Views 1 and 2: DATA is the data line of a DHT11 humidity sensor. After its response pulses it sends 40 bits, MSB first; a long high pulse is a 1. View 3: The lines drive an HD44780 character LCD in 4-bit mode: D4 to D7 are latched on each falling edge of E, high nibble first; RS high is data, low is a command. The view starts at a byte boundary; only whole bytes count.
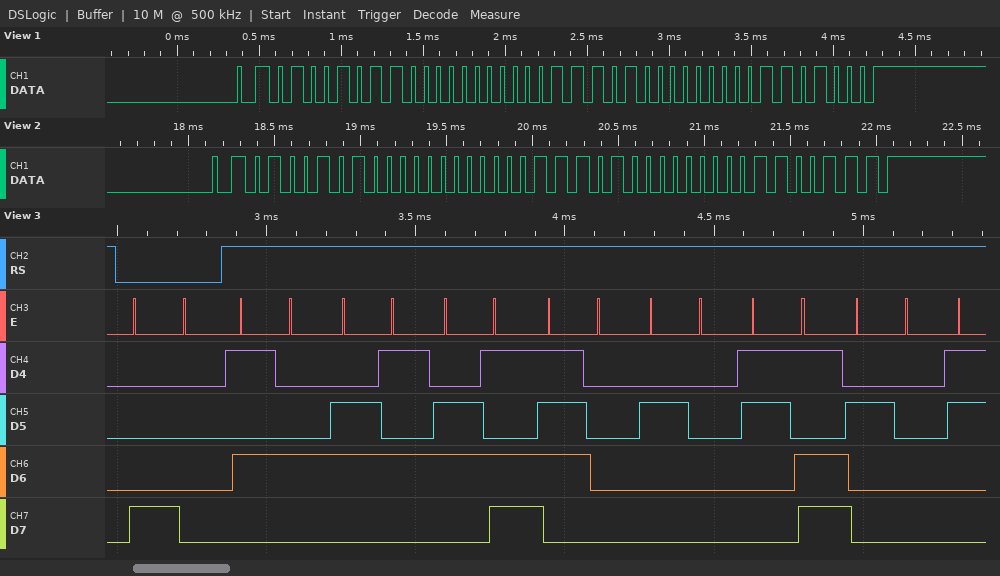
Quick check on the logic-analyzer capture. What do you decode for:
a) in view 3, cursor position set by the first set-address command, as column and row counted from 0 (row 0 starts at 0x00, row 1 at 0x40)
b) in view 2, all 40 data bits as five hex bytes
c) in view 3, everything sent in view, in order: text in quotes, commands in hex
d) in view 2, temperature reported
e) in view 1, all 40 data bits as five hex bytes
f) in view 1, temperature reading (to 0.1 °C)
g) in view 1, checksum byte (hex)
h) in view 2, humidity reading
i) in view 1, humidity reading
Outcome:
column 0, row 0
4A 00 1D 00 67
0x80 "Temp = "
29.0 °C
4B 00 1D 00 68
29.0 °C
0x68
74 %
75 %
